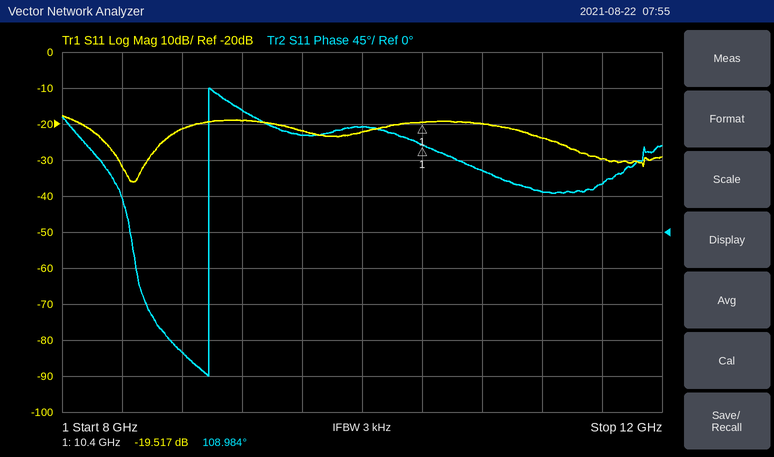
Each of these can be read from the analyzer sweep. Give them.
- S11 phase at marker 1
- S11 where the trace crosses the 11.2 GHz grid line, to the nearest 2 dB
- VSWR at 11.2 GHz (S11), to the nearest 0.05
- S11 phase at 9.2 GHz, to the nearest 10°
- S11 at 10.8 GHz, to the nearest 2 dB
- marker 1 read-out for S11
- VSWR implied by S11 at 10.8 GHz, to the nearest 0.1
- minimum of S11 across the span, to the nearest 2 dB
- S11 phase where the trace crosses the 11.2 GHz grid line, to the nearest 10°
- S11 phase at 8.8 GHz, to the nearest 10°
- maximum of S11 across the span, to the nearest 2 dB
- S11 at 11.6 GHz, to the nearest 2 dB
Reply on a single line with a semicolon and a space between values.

108.984°; -24 dB; 1.15; 150°; -20 dB; -19.517 dB; 1.2; -36 dB; 50°; -150°; -18 dB; -30 dB
